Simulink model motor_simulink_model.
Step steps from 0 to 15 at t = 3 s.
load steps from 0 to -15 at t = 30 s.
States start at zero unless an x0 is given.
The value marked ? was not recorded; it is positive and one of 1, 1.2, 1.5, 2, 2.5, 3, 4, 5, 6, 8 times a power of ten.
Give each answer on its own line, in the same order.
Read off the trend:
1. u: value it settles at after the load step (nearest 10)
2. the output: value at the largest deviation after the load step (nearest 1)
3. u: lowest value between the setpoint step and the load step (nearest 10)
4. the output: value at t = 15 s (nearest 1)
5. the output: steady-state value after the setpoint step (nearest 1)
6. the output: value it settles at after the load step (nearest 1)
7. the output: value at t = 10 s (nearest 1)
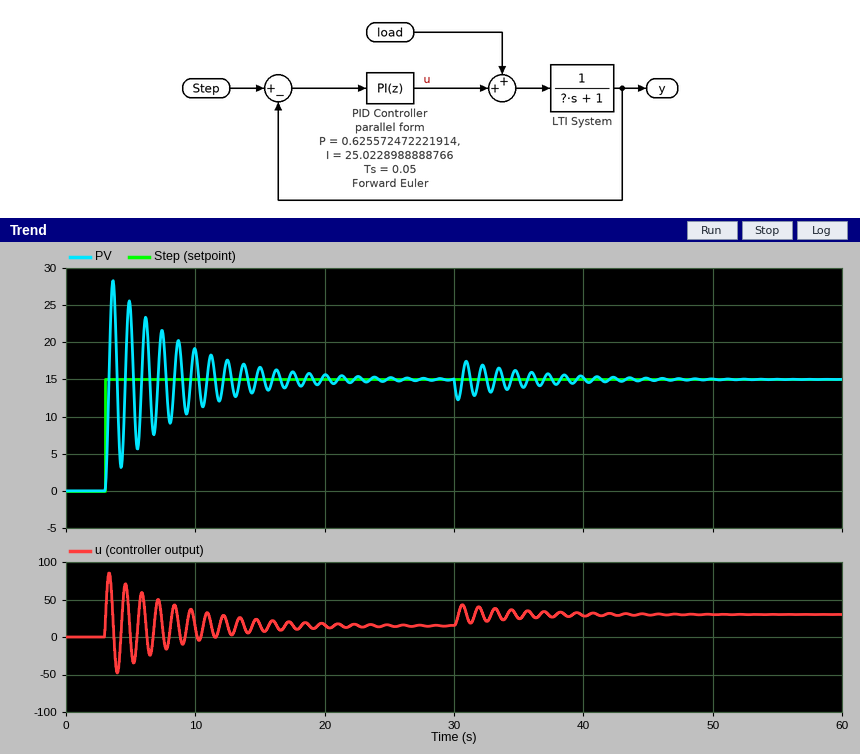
30
12
-50
17
15
15
19
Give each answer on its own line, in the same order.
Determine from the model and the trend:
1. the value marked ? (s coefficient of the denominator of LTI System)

1
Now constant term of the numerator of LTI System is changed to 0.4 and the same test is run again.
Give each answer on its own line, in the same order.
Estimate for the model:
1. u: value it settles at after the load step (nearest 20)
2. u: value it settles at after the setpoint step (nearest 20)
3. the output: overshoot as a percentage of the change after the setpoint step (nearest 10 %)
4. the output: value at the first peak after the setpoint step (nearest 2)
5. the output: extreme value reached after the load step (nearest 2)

60
40
70 %
26
14
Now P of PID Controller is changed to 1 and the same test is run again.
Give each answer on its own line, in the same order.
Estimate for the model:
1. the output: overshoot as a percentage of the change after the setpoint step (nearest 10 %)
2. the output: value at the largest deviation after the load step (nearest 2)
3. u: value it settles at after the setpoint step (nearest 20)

80 %
12
20
